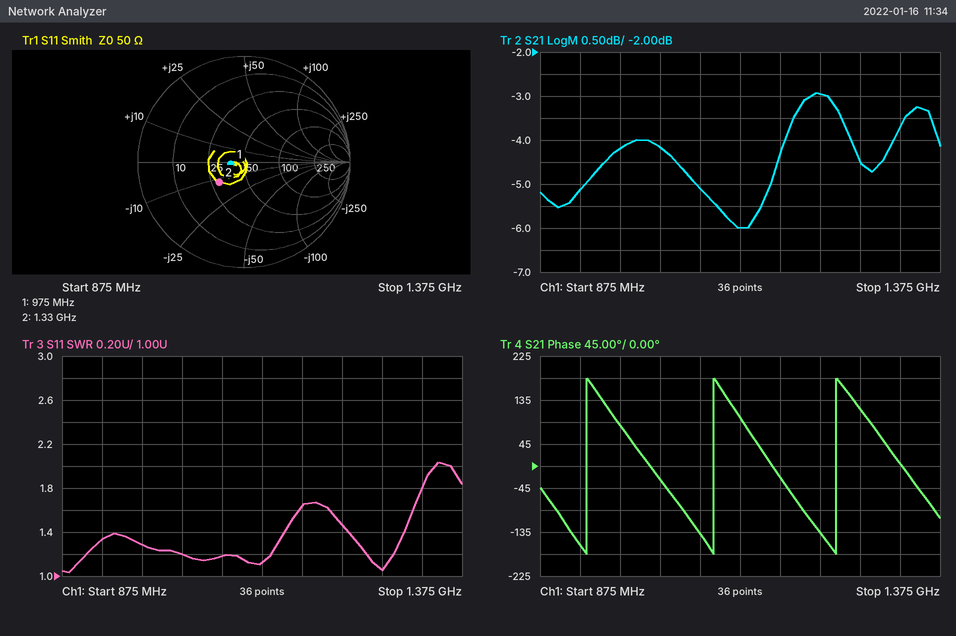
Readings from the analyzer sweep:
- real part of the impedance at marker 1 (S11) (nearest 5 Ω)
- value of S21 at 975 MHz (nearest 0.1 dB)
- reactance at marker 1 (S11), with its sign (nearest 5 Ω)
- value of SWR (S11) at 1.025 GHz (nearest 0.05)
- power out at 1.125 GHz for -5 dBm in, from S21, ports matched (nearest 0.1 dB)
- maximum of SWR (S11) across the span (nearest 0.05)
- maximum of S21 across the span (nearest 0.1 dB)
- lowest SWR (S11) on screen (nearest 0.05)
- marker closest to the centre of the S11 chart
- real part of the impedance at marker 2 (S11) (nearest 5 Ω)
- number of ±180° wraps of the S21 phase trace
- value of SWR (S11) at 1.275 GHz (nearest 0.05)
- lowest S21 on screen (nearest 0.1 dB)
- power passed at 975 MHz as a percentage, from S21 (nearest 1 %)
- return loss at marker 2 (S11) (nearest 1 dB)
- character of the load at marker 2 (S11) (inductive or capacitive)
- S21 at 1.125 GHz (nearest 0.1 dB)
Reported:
40 Ω
-4.2 dB
0 Ω
1.20
-11.0 dBm
2.05
-2.9 dB
1.05
marker 1
30 Ω
3
1.05
-6.0 dB
38 %
10 dB
capacitive
-6.0 dB
